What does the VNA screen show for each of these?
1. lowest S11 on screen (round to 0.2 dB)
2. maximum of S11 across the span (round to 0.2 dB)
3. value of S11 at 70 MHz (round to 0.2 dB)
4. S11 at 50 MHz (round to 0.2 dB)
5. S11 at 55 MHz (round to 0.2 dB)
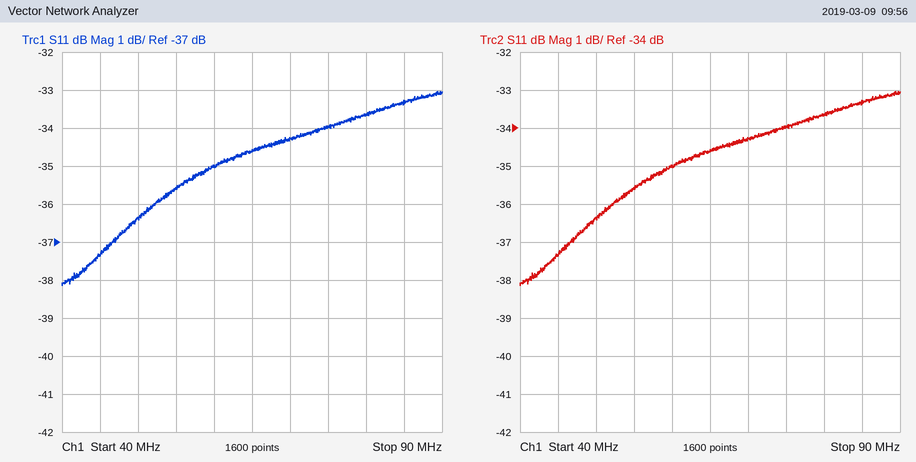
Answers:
-38.2 dB
-33.0 dB
-34.2 dB
-36.4 dB
-35.6 dB
